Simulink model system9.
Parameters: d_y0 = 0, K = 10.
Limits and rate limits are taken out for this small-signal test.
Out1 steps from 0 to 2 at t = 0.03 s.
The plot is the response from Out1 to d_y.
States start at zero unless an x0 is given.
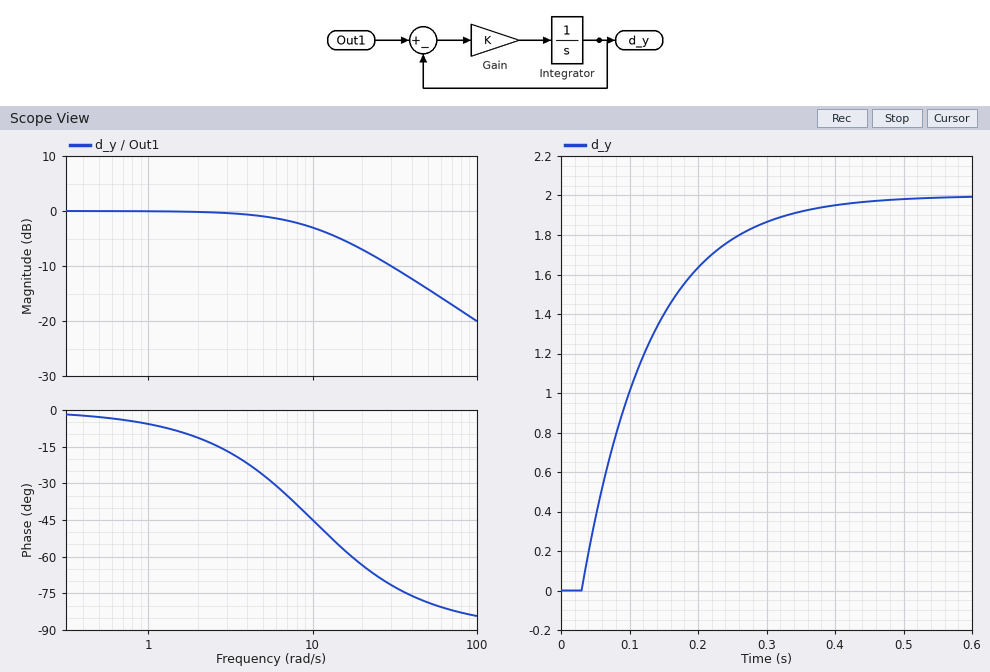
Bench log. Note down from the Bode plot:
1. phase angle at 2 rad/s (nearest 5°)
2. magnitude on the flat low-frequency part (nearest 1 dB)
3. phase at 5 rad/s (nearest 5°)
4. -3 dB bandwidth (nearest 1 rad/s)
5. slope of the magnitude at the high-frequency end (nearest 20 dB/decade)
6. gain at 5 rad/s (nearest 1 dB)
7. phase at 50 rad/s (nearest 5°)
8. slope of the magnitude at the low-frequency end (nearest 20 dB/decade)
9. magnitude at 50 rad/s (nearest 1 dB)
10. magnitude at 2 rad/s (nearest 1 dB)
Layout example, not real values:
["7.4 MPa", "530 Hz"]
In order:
["-10°", "0 dB", "-25°", "10 rad/s", "-20 dB/decade", "-1 dB", "-80°", "0 dB/decade", "-14 dB", "0 dB"]
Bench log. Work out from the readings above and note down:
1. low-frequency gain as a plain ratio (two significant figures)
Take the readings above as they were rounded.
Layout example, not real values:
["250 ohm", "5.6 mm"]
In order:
["1.0"]
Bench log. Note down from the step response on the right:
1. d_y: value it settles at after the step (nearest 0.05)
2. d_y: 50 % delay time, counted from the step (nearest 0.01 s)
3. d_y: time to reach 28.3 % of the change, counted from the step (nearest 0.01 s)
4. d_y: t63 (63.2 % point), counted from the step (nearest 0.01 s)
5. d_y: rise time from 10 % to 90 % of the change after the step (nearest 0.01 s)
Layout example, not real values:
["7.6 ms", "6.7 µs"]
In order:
["2.00", "0.07 s", "0.03 s", "0.10 s", "0.22 s"]
